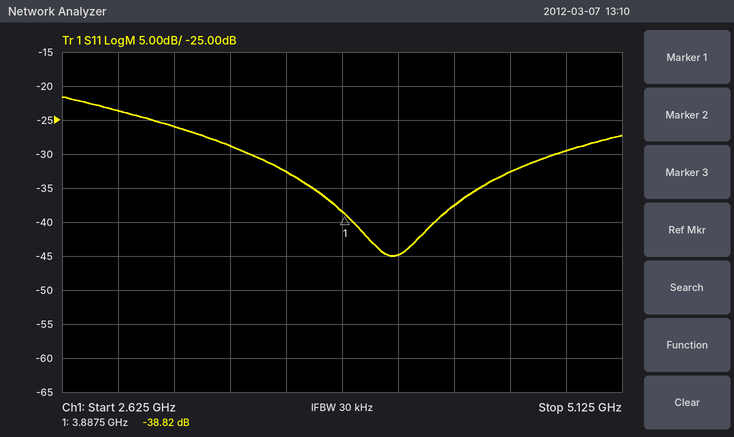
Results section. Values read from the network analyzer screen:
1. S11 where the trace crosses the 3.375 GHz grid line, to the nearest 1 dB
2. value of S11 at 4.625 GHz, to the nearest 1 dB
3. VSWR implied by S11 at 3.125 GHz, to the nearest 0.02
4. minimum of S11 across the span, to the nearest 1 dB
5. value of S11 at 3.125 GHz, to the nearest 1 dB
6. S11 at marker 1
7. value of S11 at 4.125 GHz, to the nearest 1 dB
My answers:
-29 dB
-33 dB
1.10
-45 dB
-26 dB
-38.82 dB
-45 dB
